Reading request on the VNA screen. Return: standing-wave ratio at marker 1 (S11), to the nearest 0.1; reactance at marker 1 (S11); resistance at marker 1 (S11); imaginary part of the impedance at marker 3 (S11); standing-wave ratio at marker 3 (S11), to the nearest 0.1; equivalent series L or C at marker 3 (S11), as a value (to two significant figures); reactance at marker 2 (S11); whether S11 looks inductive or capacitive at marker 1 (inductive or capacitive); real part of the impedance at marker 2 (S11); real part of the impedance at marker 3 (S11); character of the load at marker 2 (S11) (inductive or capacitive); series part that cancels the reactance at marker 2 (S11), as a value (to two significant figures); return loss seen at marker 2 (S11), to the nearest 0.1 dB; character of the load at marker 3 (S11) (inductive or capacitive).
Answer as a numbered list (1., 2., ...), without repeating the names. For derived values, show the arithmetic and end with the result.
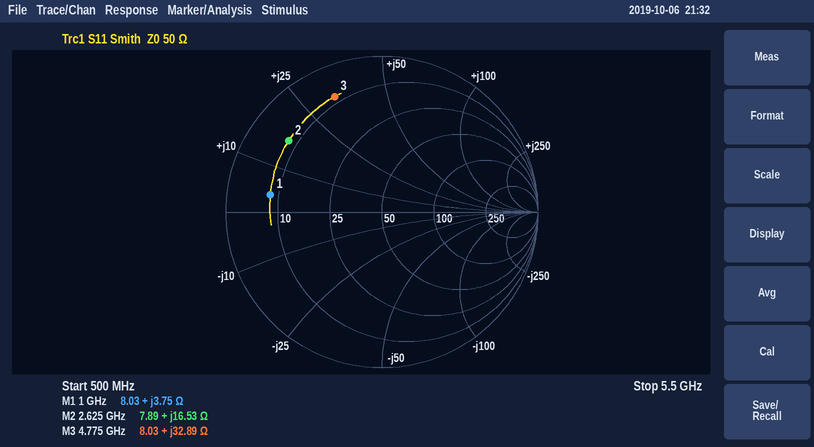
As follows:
1. 6.3
2. +3.75 Ω
3. 8.03 Ω
4. +32.89 Ω
5. 9.0
6. L = 32.89 Ω/(2π × 4.775 GHz) ≈ 1.1 nH
7. +16.53 Ω
8. inductive
9. 7.89 Ω
10. 8.03 Ω
11. inductive
12. C = 1/(2π × 2.625 GHz × 16.53 Ω) ≈ 3.7 pF
13. 2.5 dB
14. inductive
